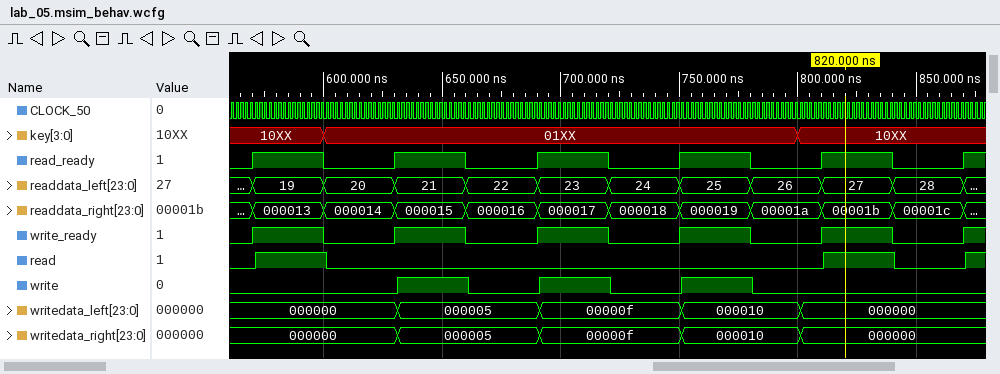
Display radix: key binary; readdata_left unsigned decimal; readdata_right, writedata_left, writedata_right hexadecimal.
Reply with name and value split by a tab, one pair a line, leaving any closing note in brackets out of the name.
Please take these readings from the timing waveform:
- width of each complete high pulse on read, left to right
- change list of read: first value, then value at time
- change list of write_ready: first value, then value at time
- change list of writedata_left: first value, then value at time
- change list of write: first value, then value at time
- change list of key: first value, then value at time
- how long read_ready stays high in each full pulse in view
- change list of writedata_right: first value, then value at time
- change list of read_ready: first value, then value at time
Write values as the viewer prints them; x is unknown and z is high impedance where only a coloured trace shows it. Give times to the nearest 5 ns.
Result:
width of each complete high pulse on read, left to right	30 ns, 30 ns
change list of read: first value, then value at time	0, 1 at 570 ns, 0 at 600 ns, 1 at 810 ns, 0 at 840 ns, 1 at 870 ns
change list of write_ready: first value, then value at time	0, 1 at 570 ns, 0 at 600 ns, 1 at 630 ns, 0 at 660 ns, 1 at 690 ns, 0 at 720 ns, 1 at 750 ns, 0 at 780 ns, 1 at 810 ns, 0 at 840 ns, 1 at 870 ns
change list of writedata_left: first value, then value at time	000000, 000005 at 630 ns, 00000f at 690 ns, 000010 at 750 ns, 000000 at 800 ns
change list of write: first value, then value at time	0, 1 at 630 ns, 0 at 660 ns, 1 at 690 ns, 0 at 720 ns, 1 at 750 ns, 0 at 780 ns
change list of key: first value, then value at time	10XX, 01XX at 600 ns, 10XX at 800 ns
how long read_ready stays high in each full pulse in view	30 ns, 30 ns, 30 ns, 30 ns, 30 ns
change list of writedata_right: first value, then value at time	000000, 000005 at 630 ns, 00000f at 690 ns, 000010 at 750 ns, 000000 at 800 ns
change list of read_ready: first value, then value at time	0, 1 at 570 ns, 0 at 600 ns, 1 at 630 ns, 0 at 660 ns, 1 at 690 ns, 0 at 720 ns, 1 at 750 ns, 0 at 780 ns, 1 at 810 ns, 0 at 840 ns, 1 at 870 ns
